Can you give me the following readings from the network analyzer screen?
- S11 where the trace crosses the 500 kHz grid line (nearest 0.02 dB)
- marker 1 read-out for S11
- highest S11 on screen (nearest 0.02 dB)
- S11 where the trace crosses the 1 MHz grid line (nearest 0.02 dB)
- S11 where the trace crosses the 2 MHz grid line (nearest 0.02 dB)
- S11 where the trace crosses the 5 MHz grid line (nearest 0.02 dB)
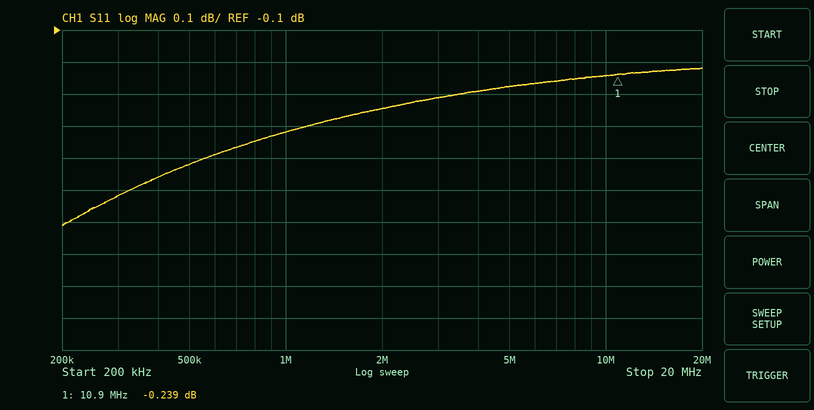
-0.52 dB
-0.239 dB
-0.22 dB
-0.42 dB
-0.34 dB
-0.28 dB
